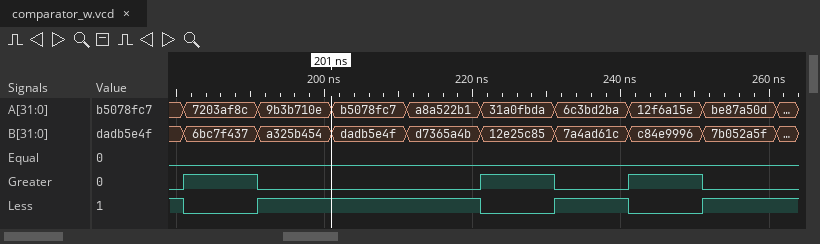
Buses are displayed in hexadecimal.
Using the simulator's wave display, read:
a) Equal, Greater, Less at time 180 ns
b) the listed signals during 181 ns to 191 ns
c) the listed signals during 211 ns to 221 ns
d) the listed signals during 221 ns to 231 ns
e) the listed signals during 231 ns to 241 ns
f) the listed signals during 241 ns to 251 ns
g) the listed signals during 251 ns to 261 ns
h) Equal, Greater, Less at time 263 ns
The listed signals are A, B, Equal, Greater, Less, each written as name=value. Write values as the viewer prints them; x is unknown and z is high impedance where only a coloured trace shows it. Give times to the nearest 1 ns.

Equal=0, Greater=0, Less=1
A=7203af8c, B=6bc7f437, Equal=0, Greater=1, Less=0
A=a8a522b1, B=d7365a4b, Equal=0, Greater=0, Less=1
A=31a0fbda, B=12e25c85, Equal=0, Greater=1, Less=0
A=6c3bd2ba, B=7a4ad61c, Equal=0, Greater=0, Less=1
A=12f6a15e, B=c84e9996, Equal=0, Greater=1, Less=0
A=be87a50d, B=7b052a5f, Equal=0, Greater=0, Less=1
Equal=0, Greater=0, Less=1
